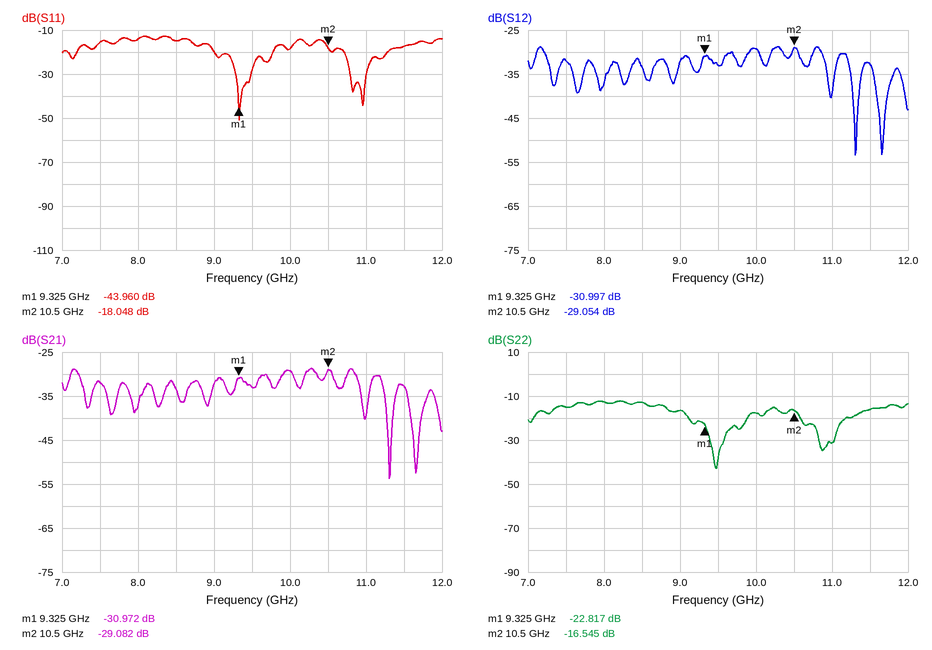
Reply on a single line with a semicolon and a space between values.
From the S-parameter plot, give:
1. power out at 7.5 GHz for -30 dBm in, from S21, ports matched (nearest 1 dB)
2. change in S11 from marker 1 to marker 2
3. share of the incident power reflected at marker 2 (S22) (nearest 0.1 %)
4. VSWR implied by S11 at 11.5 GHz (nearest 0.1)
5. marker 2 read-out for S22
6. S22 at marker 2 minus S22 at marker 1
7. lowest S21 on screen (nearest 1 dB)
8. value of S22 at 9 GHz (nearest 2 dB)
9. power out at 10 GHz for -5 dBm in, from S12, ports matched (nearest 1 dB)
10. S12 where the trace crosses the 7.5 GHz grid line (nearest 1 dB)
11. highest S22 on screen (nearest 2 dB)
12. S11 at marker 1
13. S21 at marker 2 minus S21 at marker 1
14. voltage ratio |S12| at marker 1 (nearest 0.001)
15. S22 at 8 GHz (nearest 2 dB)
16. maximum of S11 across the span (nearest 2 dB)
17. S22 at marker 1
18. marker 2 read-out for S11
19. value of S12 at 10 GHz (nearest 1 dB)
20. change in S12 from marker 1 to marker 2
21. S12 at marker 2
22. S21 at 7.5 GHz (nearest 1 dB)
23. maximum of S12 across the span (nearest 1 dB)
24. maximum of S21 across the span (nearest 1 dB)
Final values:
-62 dBm; 25.912 dB; 2.2 %; 1.3; -16.545 dB; 6.272 dB; -54 dB; -16 dB; -34 dBm; -32 dB; -12 dB; -43.960 dB; 1.890 dB; 0.028; -12 dB; -12 dB; -22.817 dB; -18.048 dB; -29 dB; 1.943 dB; -29.054 dB; -32 dB; -29 dB; -29 dB
